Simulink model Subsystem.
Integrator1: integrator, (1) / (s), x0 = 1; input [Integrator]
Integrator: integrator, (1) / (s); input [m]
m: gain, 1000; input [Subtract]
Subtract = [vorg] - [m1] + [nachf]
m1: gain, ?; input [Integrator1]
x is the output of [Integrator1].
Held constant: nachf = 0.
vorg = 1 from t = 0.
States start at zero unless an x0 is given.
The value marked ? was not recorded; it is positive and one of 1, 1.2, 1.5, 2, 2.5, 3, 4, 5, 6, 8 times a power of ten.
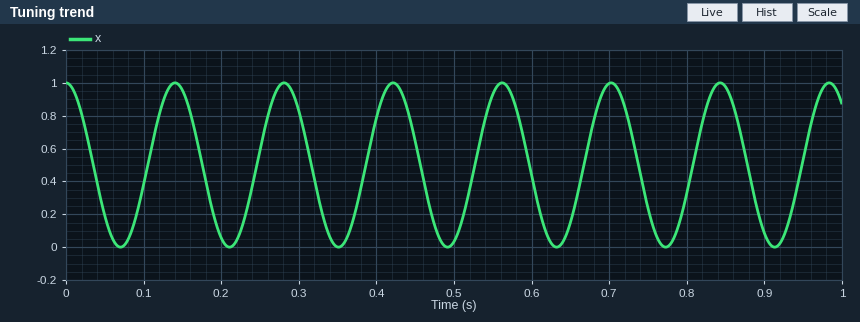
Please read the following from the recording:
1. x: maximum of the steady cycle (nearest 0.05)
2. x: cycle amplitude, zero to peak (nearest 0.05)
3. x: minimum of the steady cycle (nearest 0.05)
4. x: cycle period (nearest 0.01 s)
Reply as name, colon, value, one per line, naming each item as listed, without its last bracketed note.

x: maximum of the steady cycle: 1.00
x: cycle amplitude, zero to peak: 0.50
x: minimum of the steady cycle: 0.00
x: cycle period: 0.14 s
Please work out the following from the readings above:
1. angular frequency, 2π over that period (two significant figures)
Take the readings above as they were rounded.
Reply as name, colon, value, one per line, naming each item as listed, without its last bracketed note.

angular frequency, 2π over that period: 45 rad/s
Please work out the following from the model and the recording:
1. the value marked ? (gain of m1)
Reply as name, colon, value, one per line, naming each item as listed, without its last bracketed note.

the value marked ?: 2
